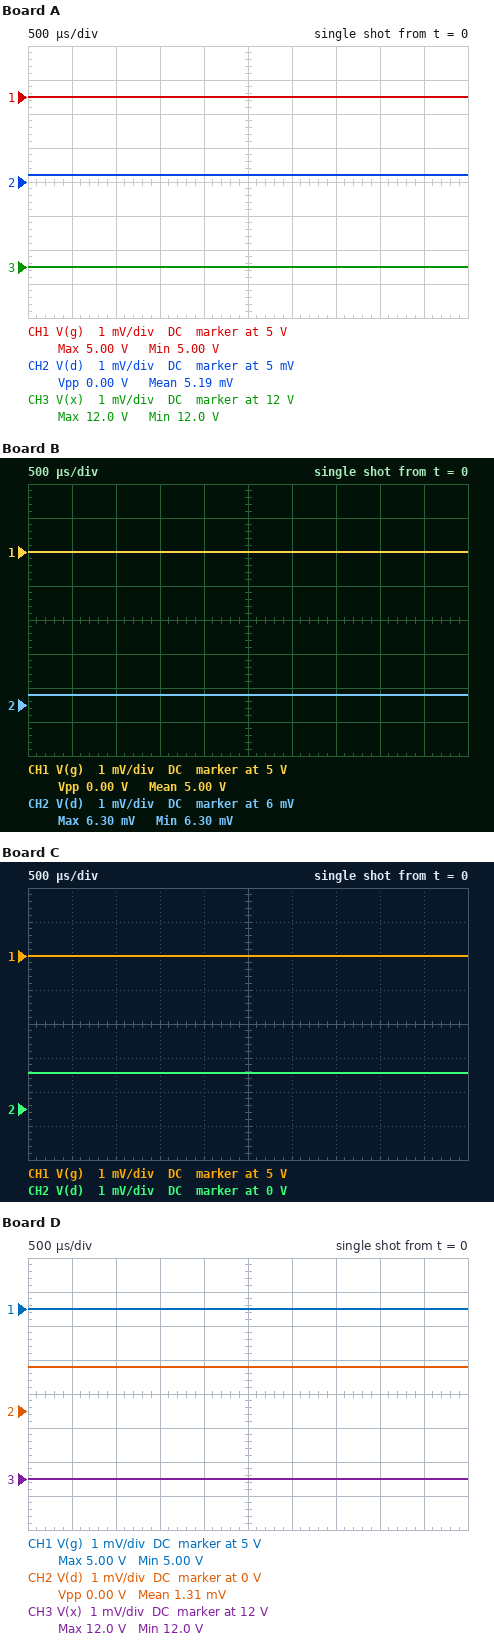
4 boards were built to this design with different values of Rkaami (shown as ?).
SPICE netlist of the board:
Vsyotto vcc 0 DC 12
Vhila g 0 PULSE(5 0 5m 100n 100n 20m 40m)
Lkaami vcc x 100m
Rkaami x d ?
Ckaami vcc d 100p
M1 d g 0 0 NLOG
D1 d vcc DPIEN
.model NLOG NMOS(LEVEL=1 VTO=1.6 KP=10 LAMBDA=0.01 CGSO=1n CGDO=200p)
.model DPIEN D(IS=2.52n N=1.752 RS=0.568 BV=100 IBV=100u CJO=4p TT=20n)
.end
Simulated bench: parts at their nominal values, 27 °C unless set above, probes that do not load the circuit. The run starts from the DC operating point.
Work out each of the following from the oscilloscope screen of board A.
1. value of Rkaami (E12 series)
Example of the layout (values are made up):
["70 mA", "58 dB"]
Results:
["68 Ω"]
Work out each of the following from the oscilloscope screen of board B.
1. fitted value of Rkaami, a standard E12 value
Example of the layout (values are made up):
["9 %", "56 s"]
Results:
["56 Ω"]
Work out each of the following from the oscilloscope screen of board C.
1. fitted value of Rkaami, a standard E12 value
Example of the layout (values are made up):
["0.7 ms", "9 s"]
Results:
["330 Ω"]
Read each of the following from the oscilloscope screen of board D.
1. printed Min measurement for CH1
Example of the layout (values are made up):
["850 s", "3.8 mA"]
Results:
["5.00 V"]
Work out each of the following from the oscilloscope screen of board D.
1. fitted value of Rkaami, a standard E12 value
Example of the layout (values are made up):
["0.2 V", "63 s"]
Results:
["270 Ω"]
